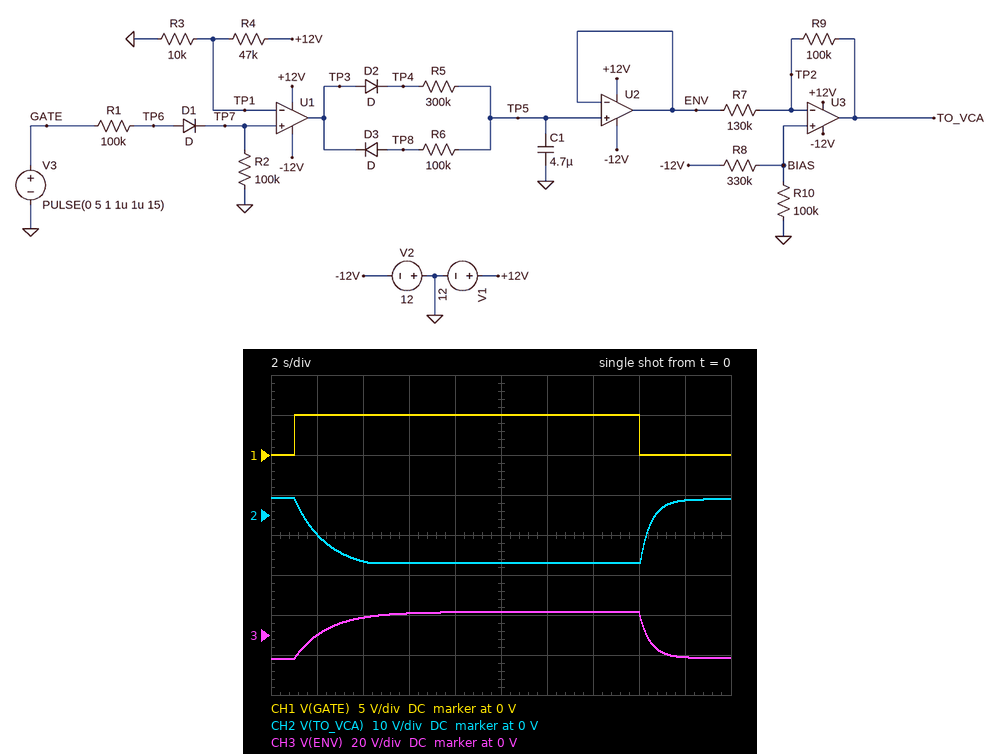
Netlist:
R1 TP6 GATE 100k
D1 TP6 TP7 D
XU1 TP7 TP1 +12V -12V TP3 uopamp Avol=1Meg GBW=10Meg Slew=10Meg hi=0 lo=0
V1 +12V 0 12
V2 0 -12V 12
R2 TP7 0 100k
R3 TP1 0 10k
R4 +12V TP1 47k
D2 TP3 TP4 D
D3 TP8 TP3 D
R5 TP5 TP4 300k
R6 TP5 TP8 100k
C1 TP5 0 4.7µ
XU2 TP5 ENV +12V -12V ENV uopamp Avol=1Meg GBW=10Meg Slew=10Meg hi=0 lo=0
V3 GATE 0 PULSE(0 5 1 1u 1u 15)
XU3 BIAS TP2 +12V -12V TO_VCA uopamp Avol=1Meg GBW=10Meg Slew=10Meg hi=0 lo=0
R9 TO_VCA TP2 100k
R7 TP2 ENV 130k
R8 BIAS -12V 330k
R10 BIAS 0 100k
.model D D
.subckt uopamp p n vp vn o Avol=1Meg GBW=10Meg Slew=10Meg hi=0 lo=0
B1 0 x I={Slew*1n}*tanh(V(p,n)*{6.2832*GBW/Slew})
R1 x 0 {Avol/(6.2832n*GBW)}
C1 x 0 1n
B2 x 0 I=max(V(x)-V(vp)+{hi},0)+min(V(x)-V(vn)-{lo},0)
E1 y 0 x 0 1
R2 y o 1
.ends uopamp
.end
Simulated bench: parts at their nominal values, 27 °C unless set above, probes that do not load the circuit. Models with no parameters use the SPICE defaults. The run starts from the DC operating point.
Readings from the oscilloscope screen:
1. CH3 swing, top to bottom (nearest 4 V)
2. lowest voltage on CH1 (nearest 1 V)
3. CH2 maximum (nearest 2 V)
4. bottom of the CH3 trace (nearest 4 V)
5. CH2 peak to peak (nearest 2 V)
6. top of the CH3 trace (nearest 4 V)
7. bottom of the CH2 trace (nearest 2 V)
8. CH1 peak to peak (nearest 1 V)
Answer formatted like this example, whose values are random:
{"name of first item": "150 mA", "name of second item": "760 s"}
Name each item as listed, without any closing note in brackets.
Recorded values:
{"CH3 swing, top to bottom": "24 V", "lowest voltage on CH1": "0 V", "CH2 maximum": "4 V", "bottom of the CH3 trace": "-12 V", "CH2 peak to peak": "16 V", "top of the CH3 trace": "12 V", "bottom of the CH2 trace": "-12 V", "CH1 peak to peak": "5 V"}
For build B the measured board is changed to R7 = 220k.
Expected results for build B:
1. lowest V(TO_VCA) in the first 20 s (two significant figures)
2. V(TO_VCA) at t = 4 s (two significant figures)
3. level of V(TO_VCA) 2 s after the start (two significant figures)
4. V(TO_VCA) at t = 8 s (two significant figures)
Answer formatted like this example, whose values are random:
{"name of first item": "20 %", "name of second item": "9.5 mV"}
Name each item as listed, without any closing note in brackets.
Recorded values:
{"lowest V(TO_VCA) in the first 20 s": "-9.3 V", "V(TO_VCA) at t = 4 s": "-8.0 V", "level of V(TO_VCA) 2 s after the start": "-4.0 V", "V(TO_VCA) at t = 8 s": "-9.2 V"}
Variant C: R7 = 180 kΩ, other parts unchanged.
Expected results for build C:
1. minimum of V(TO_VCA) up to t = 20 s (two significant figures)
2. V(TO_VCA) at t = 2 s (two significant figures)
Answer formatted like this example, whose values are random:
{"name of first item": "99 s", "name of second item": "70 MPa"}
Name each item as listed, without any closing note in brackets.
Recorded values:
{"minimum of V(TO_VCA) up to t = 20 s": "-11 V", "V(TO_VCA) at t = 2 s": "-4.3 V"}
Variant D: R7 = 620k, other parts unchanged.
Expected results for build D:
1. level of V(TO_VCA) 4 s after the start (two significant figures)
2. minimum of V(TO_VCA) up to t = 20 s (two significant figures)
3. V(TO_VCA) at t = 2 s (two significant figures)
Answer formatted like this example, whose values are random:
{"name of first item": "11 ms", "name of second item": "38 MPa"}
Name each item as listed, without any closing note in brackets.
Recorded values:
{"level of V(TO_VCA) 4 s after the start": "-4.6 V", "minimum of V(TO_VCA) up to t = 20 s": "-5.1 V", "V(TO_VCA) at t = 2 s": "-3.2 V"}
